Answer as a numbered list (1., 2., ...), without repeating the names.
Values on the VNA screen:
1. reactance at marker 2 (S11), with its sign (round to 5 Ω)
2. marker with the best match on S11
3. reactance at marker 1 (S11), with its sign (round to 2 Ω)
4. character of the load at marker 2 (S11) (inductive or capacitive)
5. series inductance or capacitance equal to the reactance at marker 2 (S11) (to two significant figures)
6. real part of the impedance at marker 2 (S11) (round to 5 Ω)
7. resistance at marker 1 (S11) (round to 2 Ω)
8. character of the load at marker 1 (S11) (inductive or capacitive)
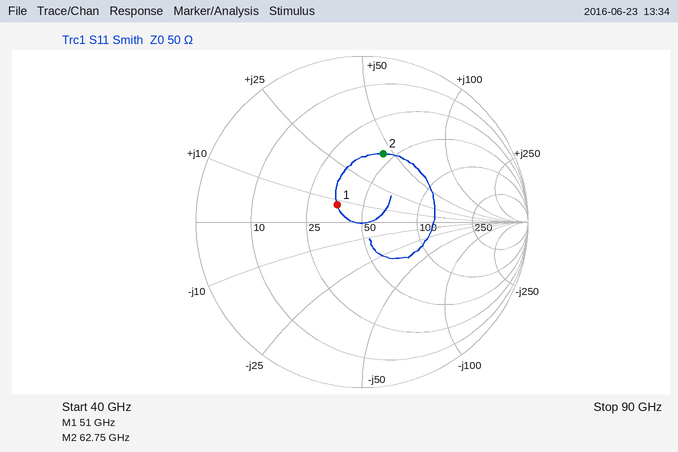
1. +45 Ω
2. marker 1
3. +8 Ω
4. inductive
5. 110 pH
6. 45 Ω
7. 36 Ω
8. inductive
